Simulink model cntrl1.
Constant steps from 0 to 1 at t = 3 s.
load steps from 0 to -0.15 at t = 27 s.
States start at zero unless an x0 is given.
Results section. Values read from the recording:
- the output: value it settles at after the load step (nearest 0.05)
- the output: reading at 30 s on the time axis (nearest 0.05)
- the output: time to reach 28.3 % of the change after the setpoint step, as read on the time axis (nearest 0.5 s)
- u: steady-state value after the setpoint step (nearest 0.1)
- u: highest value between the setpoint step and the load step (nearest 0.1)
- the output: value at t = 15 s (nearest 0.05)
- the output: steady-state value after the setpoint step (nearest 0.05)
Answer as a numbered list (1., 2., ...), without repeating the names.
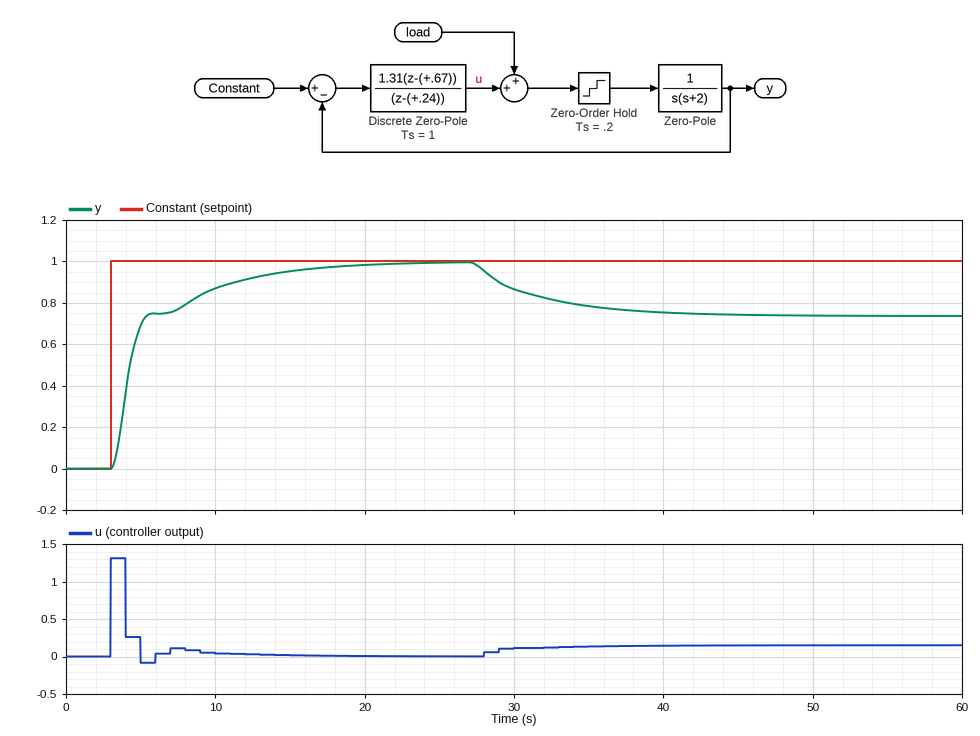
1. 0.75
2. 0.85
3. 4.0 s
4. 0.0
5. 1.3
6. 0.95
7. 1.00
